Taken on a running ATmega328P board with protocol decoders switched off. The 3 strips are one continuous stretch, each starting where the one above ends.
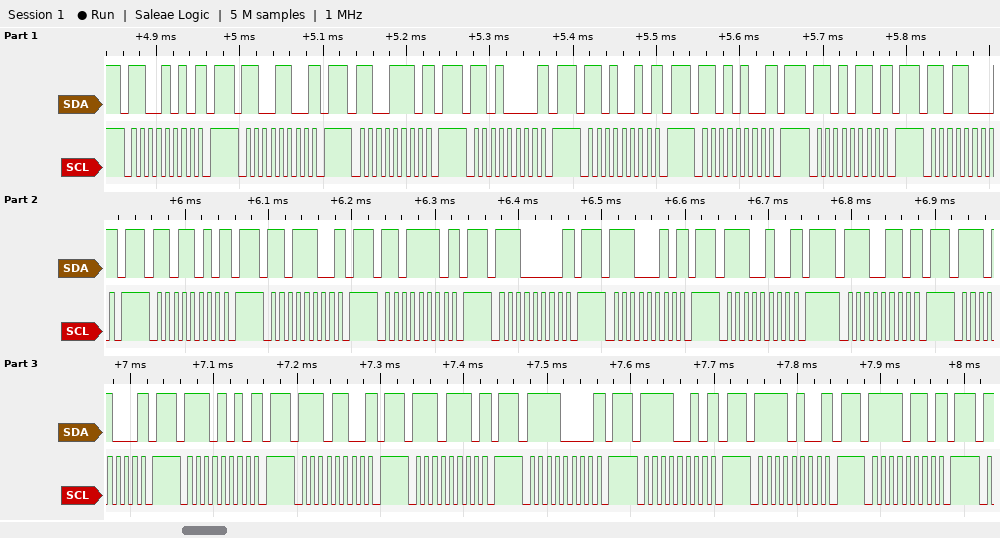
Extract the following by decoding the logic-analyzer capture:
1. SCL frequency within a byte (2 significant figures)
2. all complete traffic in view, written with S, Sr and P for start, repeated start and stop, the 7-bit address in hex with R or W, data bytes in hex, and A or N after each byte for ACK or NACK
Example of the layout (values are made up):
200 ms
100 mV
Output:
100 kHz
S 65W N P S 66W N P S 67W N P S 68W N P S 69W N P S 6AW N P S 6BW N P S 6CW N P S 6DW N P S 6EW N P S 6FW N P S 70W N P S 71W N P S 72W N P S 73W N P S 74W N P S 75W N P S 76W N P S 77W N P S 78W N P S 79W N P S 7AW N P S 7BW N P
